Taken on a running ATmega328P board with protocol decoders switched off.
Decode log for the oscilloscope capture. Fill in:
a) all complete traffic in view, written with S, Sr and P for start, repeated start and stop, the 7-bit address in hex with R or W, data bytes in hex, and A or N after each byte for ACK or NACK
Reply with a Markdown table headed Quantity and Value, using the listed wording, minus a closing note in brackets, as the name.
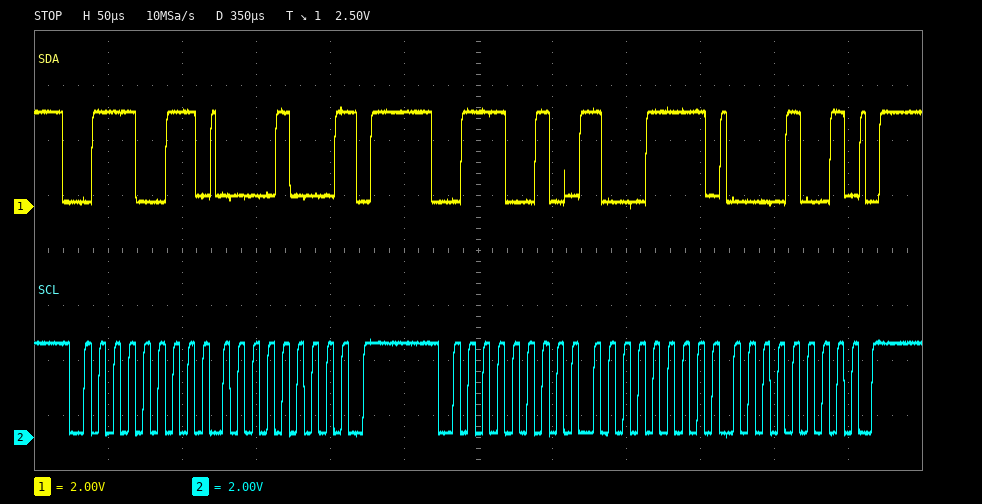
| Quantity | Value |
|---|---|
| all complete traffic in view, written with S, Sr and P for start, repeated start and stop, the 7-bit address in hex with R or W, data bytes in hex, and A or N after each byte for ACK or NACK | S 39R A 08 N P S 39W A 8F A 09 A P |
